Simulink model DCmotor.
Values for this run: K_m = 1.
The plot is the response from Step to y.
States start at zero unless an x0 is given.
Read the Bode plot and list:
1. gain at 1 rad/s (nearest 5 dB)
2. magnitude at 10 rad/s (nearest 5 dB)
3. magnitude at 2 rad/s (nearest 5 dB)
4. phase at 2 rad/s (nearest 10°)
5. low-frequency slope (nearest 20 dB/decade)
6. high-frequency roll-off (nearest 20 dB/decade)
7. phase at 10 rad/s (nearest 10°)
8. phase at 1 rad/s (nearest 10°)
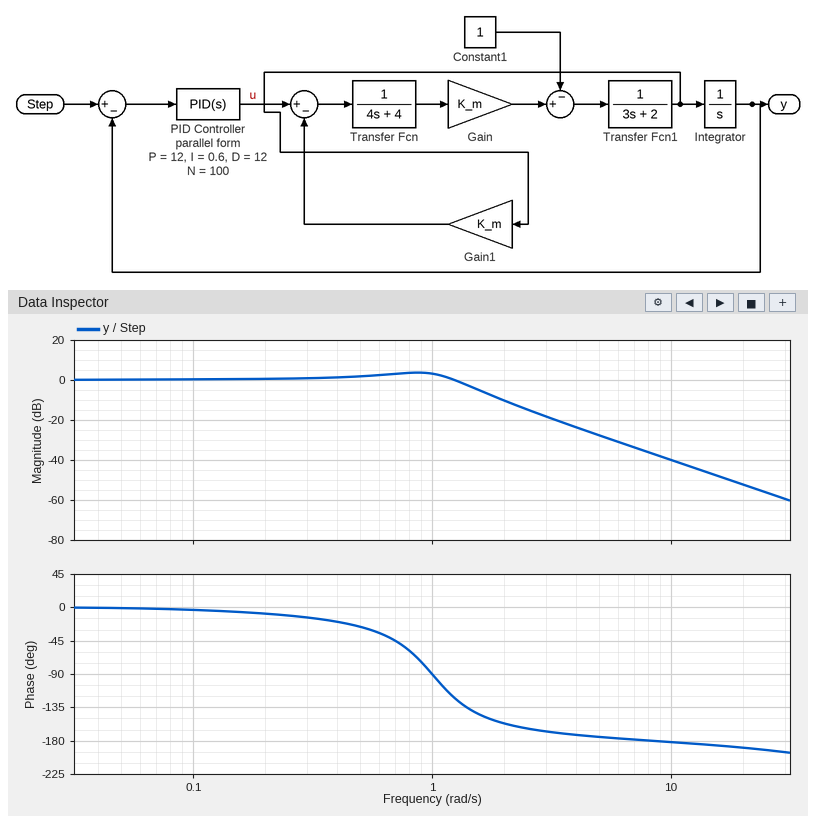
5 dB
-40 dB
-10 dB
-160°
0 dB/decade
-40 dB/decade
-180°
-90°
